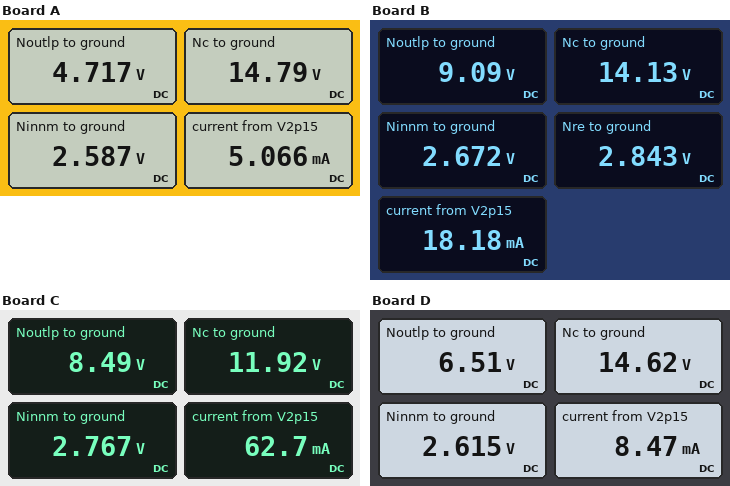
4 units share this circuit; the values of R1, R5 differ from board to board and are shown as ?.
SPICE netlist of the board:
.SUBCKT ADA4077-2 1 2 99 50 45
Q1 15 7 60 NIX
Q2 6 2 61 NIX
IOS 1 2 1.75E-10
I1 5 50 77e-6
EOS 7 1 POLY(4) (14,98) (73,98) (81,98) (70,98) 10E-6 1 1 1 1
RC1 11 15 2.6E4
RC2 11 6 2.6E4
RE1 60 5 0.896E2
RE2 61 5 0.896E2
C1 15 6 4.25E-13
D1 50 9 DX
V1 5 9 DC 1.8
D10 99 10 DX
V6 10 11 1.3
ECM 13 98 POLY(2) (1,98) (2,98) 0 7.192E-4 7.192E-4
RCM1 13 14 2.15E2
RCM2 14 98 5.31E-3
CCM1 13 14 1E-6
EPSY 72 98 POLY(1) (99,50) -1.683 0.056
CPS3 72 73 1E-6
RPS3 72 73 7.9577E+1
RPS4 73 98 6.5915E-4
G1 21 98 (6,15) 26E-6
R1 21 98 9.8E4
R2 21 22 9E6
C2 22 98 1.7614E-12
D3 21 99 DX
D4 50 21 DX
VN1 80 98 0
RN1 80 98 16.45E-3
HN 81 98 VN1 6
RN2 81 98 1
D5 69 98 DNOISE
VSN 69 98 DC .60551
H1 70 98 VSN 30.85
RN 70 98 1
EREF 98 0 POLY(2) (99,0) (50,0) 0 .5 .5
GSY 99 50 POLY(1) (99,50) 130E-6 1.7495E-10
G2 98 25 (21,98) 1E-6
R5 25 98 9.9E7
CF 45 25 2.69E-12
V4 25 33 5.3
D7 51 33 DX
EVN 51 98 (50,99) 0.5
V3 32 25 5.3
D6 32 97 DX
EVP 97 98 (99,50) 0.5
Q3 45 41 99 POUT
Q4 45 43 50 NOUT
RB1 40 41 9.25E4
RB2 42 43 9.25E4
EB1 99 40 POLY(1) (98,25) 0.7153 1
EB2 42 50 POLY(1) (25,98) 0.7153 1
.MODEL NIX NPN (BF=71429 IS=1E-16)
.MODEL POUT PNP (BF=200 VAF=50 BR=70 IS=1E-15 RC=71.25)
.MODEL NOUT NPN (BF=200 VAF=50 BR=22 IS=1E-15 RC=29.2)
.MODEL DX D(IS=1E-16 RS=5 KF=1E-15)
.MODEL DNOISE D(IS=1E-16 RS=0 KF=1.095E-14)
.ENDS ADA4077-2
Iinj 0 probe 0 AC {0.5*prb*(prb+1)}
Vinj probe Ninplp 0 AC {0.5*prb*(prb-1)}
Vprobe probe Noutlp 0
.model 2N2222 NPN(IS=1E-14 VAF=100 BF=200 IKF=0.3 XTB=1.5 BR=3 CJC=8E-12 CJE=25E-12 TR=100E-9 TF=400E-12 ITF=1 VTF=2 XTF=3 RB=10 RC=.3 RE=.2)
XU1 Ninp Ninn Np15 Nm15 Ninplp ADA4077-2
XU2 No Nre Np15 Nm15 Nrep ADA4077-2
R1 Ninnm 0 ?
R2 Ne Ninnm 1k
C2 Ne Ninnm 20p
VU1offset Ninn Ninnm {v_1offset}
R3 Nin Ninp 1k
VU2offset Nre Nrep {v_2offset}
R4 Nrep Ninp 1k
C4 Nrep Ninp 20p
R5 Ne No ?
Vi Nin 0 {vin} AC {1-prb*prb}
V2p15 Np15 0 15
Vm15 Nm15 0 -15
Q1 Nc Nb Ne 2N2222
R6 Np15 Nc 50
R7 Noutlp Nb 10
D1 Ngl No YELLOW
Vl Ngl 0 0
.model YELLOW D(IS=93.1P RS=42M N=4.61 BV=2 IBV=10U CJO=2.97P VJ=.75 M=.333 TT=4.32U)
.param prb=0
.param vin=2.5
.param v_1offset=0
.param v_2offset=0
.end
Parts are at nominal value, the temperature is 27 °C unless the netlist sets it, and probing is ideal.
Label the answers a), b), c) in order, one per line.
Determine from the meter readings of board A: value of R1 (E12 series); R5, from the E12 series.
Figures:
a) 1.8 kΩ
b) 470 Ω
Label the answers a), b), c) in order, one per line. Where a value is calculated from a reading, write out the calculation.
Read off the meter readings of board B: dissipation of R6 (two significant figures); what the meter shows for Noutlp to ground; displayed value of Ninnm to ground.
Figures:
a) (15 V - 14.13 V)^2 / 50 Ω = 15 mW
b) 9.09 V
c) 2.672 V
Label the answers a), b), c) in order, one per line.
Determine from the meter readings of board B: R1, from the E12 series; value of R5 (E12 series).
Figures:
a) 470 Ω
b) 470 Ω
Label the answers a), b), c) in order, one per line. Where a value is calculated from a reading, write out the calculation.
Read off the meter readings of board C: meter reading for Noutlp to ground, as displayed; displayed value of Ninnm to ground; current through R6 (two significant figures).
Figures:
a) 8.49 V
b) 2.767 V
c) (15 V - 11.92 V) / 50 Ω = 62 mA
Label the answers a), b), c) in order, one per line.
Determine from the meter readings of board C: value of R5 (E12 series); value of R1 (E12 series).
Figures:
a) 82 Ω
b) 560 Ω
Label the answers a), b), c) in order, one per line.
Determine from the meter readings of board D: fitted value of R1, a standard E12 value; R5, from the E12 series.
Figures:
a) 820 Ω
b) 680 Ω
